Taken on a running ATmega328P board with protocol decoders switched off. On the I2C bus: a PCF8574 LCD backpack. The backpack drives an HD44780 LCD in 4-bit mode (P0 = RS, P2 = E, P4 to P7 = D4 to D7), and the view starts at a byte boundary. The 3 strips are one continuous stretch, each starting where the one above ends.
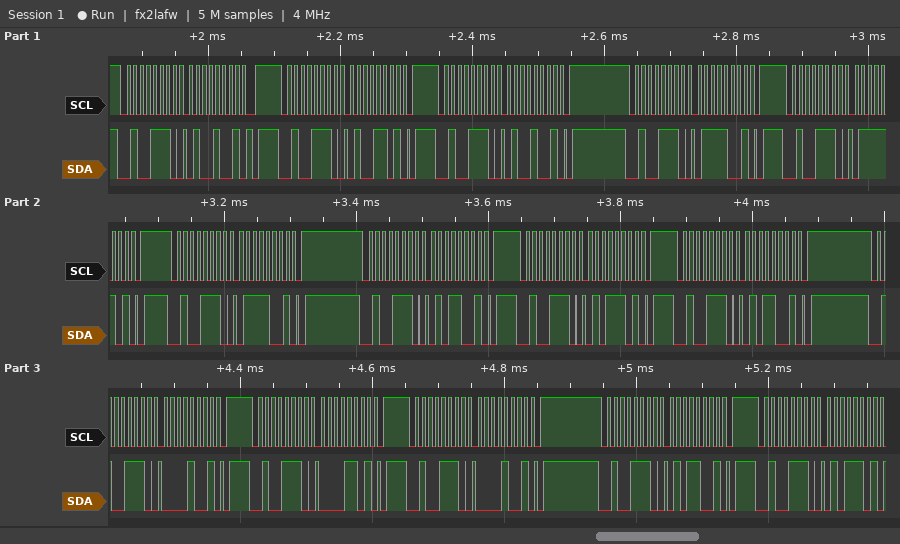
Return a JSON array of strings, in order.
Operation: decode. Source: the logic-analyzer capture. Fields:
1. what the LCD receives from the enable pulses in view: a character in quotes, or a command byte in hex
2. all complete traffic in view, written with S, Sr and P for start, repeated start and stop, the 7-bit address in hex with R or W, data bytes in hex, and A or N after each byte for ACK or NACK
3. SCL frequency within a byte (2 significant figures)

["'G' 'P'", "S 27W A 49 A P S 27W A 4D A P S 27W A 49 A P S 27W A 79 A P S 27W A 7D A P S 27W A 79 A P S 27W A 59 A P S 27W A 5D A P S 27W A 59 A P S 27W A 09 A P S 27W A 0D A P S 27W A 09 A P S 27W A 59 A P S 27W A 5D A", "100 kHz"]
